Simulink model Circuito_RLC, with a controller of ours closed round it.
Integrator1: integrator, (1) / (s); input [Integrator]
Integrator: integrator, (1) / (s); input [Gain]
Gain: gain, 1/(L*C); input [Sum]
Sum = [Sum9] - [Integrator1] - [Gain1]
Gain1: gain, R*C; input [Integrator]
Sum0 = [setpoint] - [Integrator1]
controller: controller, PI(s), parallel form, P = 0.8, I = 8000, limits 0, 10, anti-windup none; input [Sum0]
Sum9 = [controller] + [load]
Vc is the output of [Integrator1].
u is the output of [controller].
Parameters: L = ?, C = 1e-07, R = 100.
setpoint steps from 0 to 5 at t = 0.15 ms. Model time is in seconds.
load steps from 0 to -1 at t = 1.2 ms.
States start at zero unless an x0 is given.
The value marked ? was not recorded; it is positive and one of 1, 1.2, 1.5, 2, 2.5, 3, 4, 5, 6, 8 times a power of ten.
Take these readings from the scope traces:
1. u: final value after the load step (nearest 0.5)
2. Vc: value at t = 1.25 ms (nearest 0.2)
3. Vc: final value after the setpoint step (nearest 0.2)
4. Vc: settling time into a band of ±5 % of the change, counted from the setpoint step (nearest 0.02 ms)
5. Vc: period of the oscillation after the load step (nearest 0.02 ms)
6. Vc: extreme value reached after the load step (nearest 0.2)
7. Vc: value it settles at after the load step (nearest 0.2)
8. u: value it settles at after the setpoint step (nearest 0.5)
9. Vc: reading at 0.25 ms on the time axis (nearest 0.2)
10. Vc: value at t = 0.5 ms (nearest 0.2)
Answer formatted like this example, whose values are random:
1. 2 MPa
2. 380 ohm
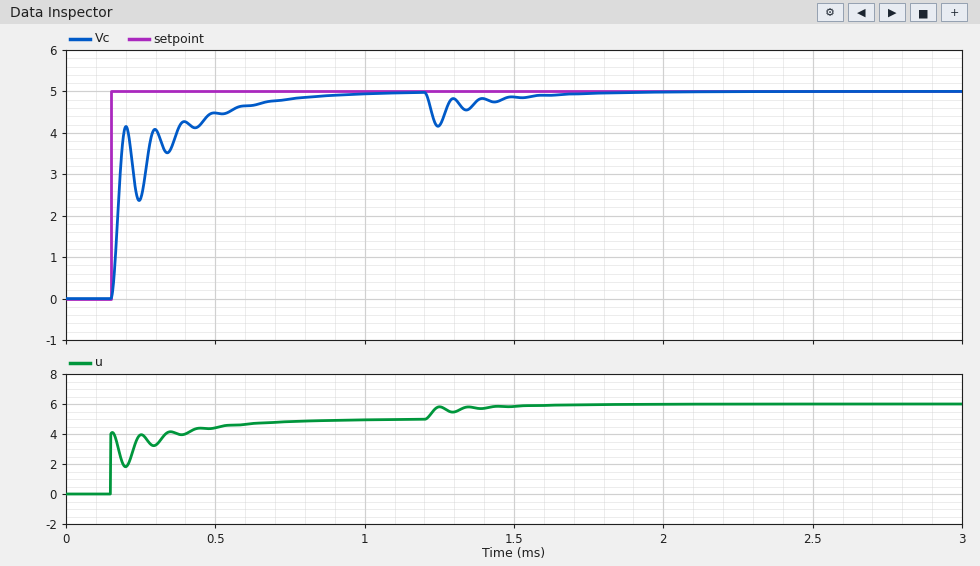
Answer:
1. 6.0
2. 4.2
3. 5.0
4. 0.52 ms
5. 0.10 ms
6. 4.2
7. 5.0
8. 5.0
9. 2.4
10. 4.4
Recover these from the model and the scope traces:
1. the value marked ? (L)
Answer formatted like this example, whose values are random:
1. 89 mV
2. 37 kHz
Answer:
1. 0.004
